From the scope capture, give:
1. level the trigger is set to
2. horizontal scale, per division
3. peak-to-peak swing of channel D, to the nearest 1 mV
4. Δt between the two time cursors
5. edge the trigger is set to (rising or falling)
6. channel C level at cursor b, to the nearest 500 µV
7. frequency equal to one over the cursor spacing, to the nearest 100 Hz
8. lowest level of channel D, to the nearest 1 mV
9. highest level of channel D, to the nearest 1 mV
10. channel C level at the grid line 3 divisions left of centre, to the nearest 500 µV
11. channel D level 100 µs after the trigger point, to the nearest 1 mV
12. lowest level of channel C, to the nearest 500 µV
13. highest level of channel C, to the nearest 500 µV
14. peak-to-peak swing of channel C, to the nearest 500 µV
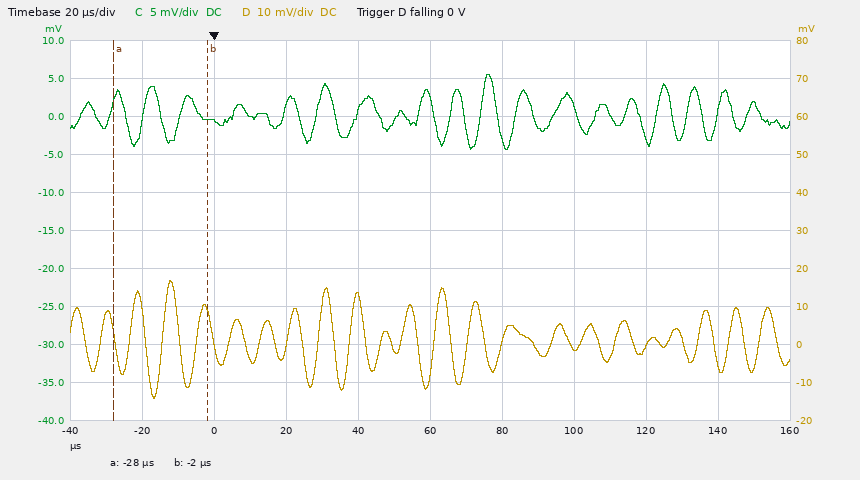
0 V
20 µs
31 mV
26 µs
falling
-500 µV
38.5 kHz
-14 mV
17 mV
-500 µV
-1 mV
-4.5 mV
5.5 mV
10.0 mV
